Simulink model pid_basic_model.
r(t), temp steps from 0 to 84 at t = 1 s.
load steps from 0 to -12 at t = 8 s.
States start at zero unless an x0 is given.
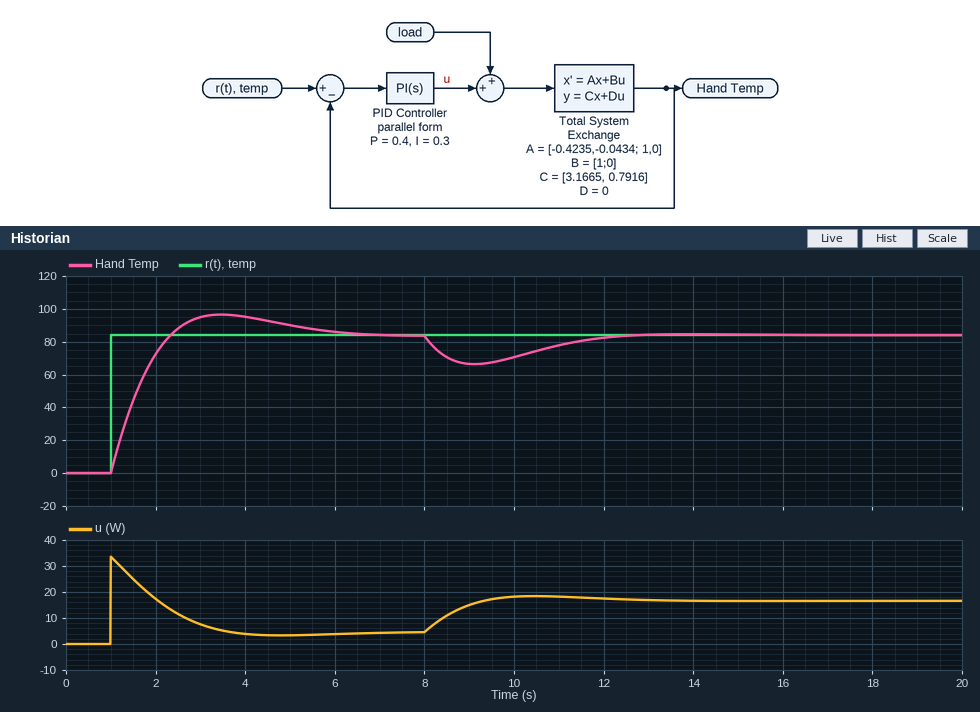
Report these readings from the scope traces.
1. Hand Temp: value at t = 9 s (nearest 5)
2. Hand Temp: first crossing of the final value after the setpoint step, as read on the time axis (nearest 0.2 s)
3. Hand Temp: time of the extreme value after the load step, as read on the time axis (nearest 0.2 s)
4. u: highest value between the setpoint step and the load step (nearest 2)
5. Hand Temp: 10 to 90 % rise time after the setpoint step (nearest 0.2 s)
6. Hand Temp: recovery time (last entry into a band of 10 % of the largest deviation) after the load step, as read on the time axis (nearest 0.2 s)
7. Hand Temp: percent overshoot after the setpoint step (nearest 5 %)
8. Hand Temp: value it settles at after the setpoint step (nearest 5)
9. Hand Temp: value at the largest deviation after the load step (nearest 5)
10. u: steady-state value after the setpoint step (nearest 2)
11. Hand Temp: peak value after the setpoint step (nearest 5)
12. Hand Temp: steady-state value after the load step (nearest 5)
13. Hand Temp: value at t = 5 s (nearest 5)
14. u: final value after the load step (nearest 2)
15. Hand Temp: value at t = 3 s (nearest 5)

65
2.4 s
9.2 s
34
1.0 s
12.0 s
15 %
85
65
4
95
85
90
16
95
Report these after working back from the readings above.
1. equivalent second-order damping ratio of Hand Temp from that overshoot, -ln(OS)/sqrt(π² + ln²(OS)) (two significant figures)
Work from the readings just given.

0.52
